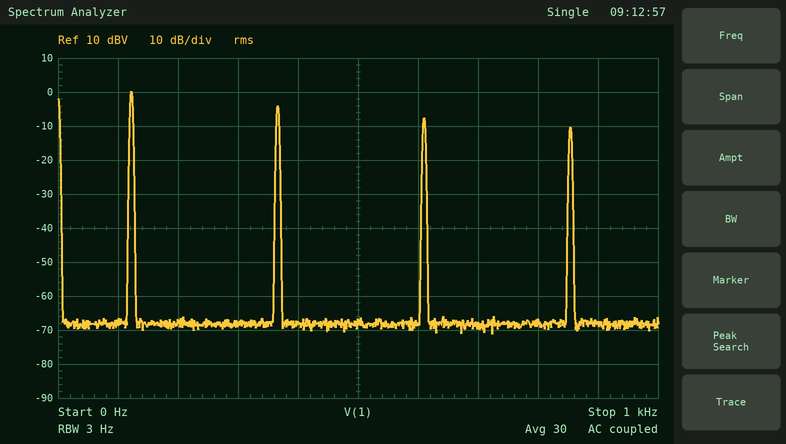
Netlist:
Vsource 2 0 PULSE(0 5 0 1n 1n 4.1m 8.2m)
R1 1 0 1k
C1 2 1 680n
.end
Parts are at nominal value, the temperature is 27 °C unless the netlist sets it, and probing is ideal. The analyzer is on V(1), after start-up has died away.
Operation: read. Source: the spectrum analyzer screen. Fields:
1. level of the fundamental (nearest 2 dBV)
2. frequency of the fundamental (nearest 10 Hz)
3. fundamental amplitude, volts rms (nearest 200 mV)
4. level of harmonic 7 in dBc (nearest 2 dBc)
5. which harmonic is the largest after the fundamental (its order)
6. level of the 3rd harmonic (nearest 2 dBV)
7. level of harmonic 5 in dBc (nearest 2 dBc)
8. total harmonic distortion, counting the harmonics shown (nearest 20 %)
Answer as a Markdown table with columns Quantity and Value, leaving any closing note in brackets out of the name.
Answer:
| Quantity | Value |
|---|---|
| level of the fundamental | 0 dBV |
| frequency of the fundamental | 120 Hz |
| fundamental amplitude, volts rms | 1.0 V |
| level of harmonic 7 in dBc | -10 dBc |
| which harmonic is the largest after the fundamental | 3 |
| level of the 3rd harmonic | -4 dBV |
| level of harmonic 5 in dBc | -8 dBc |
| total harmonic distortion, counting the harmonics shown | 80 % |
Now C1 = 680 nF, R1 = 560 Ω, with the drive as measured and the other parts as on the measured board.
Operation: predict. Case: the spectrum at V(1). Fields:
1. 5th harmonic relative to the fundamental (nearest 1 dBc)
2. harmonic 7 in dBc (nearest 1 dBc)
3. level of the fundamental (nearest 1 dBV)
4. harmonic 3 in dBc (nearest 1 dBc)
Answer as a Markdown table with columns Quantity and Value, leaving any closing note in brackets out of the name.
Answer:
| Quantity | Value |
|---|---|
| 5th harmonic relative to the fundamental | -5 dBc |
| harmonic 7 in dBc | -7 dBc |
| level of the fundamental | -4 dBV |
| harmonic 3 in dBc | -2 dBc |
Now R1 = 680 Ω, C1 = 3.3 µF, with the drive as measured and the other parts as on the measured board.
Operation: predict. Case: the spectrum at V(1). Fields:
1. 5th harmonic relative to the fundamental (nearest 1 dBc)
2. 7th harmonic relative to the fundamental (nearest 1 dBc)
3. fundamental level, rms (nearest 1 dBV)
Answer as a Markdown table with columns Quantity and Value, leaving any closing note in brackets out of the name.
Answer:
| Quantity | Value |
|---|---|
| 5th harmonic relative to the fundamental | -13 dBc |
| 7th harmonic relative to the fundamental | -16 dBc |
| fundamental level, rms | 6 dBV |
